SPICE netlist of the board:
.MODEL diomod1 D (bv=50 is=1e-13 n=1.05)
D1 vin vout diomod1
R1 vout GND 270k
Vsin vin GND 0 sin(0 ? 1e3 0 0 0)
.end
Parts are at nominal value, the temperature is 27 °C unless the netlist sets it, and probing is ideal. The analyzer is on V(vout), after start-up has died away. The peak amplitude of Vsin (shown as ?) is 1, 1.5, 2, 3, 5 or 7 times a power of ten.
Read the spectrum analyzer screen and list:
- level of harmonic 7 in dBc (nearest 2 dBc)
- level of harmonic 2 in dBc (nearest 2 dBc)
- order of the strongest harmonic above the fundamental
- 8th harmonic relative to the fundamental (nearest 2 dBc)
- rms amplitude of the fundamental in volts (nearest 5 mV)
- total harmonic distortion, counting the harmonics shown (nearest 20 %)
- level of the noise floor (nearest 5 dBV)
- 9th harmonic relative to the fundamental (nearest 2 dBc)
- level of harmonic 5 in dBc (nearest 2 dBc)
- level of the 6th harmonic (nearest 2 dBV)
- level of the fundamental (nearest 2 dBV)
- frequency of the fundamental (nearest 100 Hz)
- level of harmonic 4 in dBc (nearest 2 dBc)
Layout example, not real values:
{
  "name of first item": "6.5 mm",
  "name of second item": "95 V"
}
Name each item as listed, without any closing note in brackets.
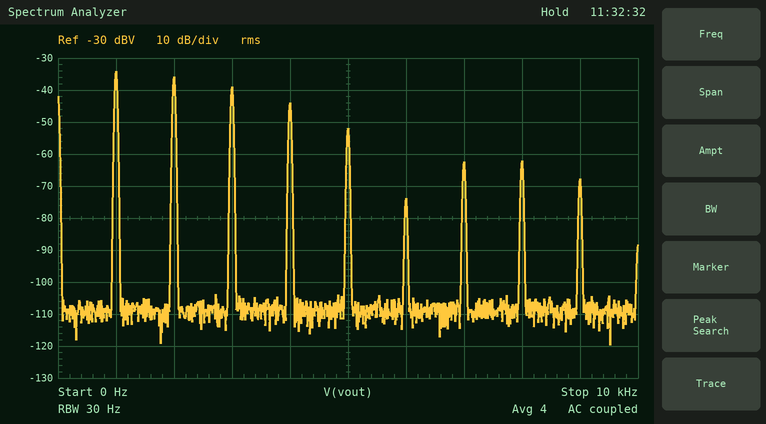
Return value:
{
  "level of harmonic 7 in dBc": "-28 dBc",
  "level of harmonic 2 in dBc": "-2 dBc",
  "order of the strongest harmonic above the fundamental": "2",
  "8th harmonic relative to the fundamental": "-28 dBc",
  "rms amplitude of the fundamental in volts": "20 mV",
  "total harmonic distortion, counting the harmonics shown": "100 %",
  "level of the noise floor": "-110 dBV",
  "9th harmonic relative to the fundamental": "-34 dBc",
  "level of harmonic 5 in dBc": "-18 dBc",
  "level of the 6th harmonic": "-74 dBV",
  "level of the fundamental": "-34 dBV",
  "frequency of the fundamental": "1.0 kHz",
  "level of harmonic 4 in dBc": "-10 dBc"
}
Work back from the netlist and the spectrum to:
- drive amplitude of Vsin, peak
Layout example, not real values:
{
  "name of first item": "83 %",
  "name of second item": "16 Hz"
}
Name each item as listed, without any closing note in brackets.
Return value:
{
  "drive amplitude of Vsin, peak": "500 mV"
}
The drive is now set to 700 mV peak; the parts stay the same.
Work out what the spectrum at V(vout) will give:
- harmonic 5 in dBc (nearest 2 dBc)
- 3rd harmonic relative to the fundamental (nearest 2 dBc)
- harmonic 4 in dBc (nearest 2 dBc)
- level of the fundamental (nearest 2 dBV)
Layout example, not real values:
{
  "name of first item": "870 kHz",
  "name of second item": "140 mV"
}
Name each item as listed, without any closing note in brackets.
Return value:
{
  "harmonic 5 in dBc": "-30 dBc",
  "3rd harmonic relative to the fundamental": "-8 dBc",
  "harmonic 4 in dBc": "-18 dBc",
  "level of the fundamental": "-24 dBV"
}
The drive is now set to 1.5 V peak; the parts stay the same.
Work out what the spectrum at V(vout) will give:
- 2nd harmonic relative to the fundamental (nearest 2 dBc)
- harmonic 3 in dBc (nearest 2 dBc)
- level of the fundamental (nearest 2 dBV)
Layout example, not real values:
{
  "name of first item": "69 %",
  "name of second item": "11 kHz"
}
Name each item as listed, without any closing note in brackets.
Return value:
{
  "2nd harmonic relative to the fundamental": "-4 dBc",
  "harmonic 3 in dBc": "-16 dBc",
  "level of the fundamental": "-10 dBV"
}
